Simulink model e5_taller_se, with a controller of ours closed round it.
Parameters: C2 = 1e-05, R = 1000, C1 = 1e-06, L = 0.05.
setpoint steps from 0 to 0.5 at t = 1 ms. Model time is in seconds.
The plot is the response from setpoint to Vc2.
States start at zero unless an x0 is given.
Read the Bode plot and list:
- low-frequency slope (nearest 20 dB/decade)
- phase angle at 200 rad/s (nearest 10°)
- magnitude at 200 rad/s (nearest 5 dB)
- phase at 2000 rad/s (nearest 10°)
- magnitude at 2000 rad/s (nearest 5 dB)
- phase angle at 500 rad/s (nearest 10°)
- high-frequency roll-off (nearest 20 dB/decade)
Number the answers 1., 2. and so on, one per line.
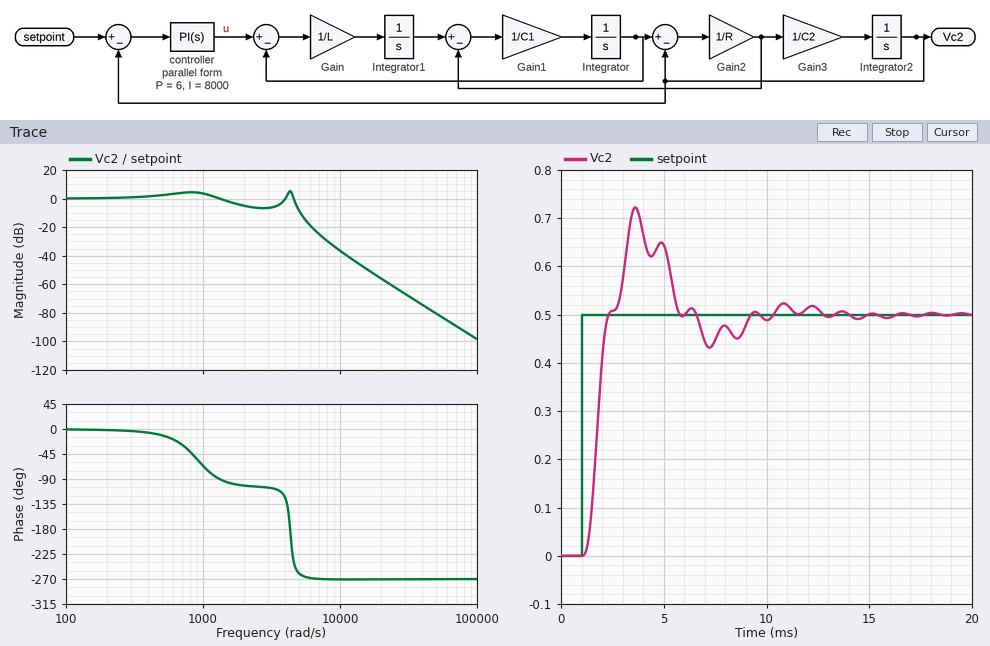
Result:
1. 0 dB/decade
2. 0°
3. 0 dB
4. -100°
5. -5 dB
6. -10°
7. -60 dB/decade
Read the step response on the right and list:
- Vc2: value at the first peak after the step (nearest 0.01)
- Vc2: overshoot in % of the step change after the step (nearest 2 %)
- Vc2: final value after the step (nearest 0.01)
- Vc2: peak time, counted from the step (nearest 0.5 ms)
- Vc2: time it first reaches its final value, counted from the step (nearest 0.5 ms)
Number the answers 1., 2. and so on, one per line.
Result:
1. 0.72
2. 44 %
3. 0.50
4. 2.5 ms
5. 1.5 ms
